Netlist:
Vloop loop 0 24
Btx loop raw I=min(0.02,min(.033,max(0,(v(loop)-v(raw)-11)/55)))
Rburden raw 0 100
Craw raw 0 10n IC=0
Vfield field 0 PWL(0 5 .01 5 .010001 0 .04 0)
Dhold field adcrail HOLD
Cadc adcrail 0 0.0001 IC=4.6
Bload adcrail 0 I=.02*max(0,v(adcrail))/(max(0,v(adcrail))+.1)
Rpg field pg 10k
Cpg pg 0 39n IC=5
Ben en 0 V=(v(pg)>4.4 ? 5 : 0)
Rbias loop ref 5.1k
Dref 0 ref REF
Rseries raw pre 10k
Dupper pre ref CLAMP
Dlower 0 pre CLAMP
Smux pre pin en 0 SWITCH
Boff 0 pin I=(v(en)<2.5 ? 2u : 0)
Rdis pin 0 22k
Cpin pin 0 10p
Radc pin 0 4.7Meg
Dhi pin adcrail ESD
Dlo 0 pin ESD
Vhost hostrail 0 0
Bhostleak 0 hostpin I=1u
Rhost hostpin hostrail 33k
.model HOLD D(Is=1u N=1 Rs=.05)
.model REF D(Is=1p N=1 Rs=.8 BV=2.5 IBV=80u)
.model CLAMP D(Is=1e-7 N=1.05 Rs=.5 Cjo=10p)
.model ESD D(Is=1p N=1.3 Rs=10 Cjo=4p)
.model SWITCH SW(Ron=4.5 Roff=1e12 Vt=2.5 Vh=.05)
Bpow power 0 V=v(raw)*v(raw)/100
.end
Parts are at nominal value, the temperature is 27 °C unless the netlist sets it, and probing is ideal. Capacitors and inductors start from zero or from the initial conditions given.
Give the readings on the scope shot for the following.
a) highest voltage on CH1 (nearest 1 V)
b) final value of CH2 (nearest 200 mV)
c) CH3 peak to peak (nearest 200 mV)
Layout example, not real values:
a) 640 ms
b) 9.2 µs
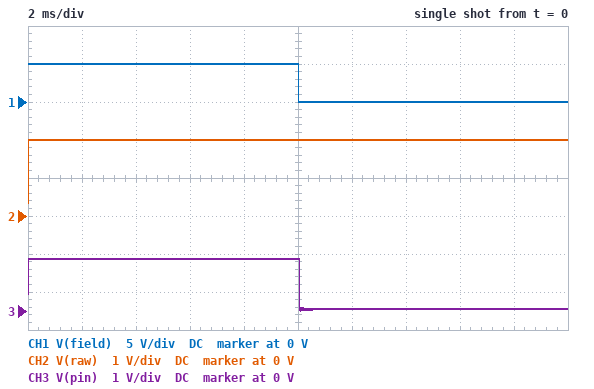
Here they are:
a) 5 V
b) 2.0 V
c) 1.4 V
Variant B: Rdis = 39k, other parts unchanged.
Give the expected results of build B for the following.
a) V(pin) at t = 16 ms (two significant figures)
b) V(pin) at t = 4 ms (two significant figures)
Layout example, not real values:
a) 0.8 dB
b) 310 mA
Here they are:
a) 77 mV
b) 1.6 V
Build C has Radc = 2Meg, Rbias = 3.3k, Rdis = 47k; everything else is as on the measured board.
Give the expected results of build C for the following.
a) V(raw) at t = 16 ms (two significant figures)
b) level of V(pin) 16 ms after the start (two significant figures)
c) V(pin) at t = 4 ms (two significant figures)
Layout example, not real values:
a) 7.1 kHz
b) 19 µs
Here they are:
a) 2.0 V
b) 92 mV
c) 1.6 V
